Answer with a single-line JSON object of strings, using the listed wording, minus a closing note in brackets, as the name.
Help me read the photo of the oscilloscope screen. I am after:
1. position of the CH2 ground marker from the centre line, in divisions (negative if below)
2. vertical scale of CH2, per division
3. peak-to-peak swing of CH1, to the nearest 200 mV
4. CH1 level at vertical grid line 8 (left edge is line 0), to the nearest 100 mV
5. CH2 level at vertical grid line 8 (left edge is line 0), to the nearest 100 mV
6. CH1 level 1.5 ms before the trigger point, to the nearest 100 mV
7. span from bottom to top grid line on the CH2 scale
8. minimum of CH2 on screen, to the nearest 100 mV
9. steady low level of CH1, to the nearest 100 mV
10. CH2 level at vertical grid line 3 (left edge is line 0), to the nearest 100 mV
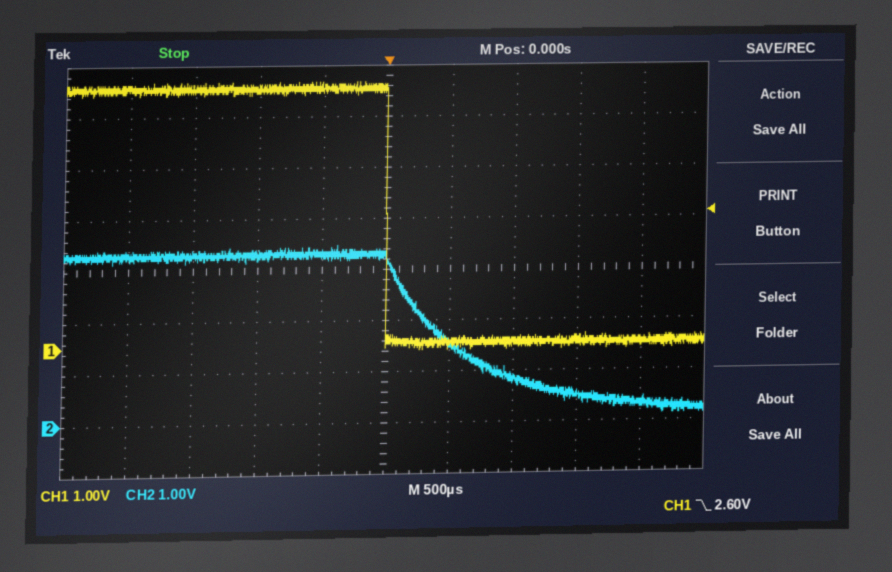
{"position of the CH2 ground marker from the centre line, in divisions": "-3.0 div", "vertical scale of CH2, per division": "1 V", "peak-to-peak swing of CH1, to the nearest 200 mV": "5.2 V", "CH1 level at vertical grid line 8 (left edge is line 0), to the nearest 100 mV": "100 mV", "CH2 level at vertical grid line 8 (left edge is line 0), to the nearest 100 mV": "500 mV", "CH1 level 1.5 ms before the trigger point, to the nearest 100 mV": "5.1 V", "span from bottom to top grid line on the CH2 scale": "8 V", "minimum of CH2 on screen, to the nearest 100 mV": "200 mV", "steady low level of CH1, to the nearest 100 mV": "100 mV", "CH2 level at vertical grid line 3 (left edge is line 0), to the nearest 100 mV": "3.3 V"}
